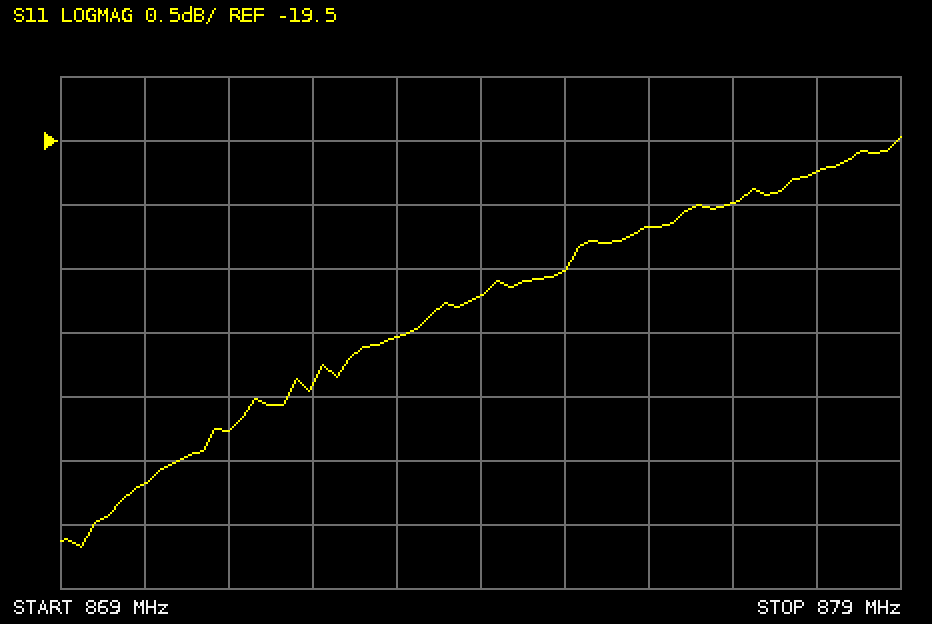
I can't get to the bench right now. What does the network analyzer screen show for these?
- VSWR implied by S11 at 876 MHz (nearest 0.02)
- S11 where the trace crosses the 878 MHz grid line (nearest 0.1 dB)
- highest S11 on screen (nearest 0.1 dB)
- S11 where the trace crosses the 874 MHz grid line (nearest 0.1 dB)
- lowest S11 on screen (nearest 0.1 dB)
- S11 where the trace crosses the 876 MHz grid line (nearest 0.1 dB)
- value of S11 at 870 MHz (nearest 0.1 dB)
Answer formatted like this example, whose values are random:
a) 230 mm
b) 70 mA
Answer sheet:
a) 1.22
b) -19.7 dB
c) -19.5 dB
d) -20.7 dB
e) -22.7 dB
f) -20.2 dB
g) -22.2 dB
